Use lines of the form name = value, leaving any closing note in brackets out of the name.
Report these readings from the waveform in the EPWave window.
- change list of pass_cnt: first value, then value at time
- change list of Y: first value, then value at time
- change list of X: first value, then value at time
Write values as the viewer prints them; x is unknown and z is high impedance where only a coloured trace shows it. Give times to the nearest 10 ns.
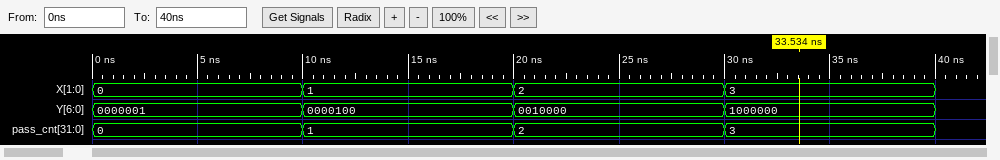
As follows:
change list of pass_cnt: first value, then value at time = 0, 1 at 10 ns, 2 at 20 ns, 3 at 30 ns
change list of Y: first value, then value at time = 0000001, 0000100 at 10 ns, 0010000 at 20 ns, 1000000 at 30 ns
change list of X: first value, then value at time = 0, 1 at 10 ns, 2 at 20 ns, 3 at 30 ns
